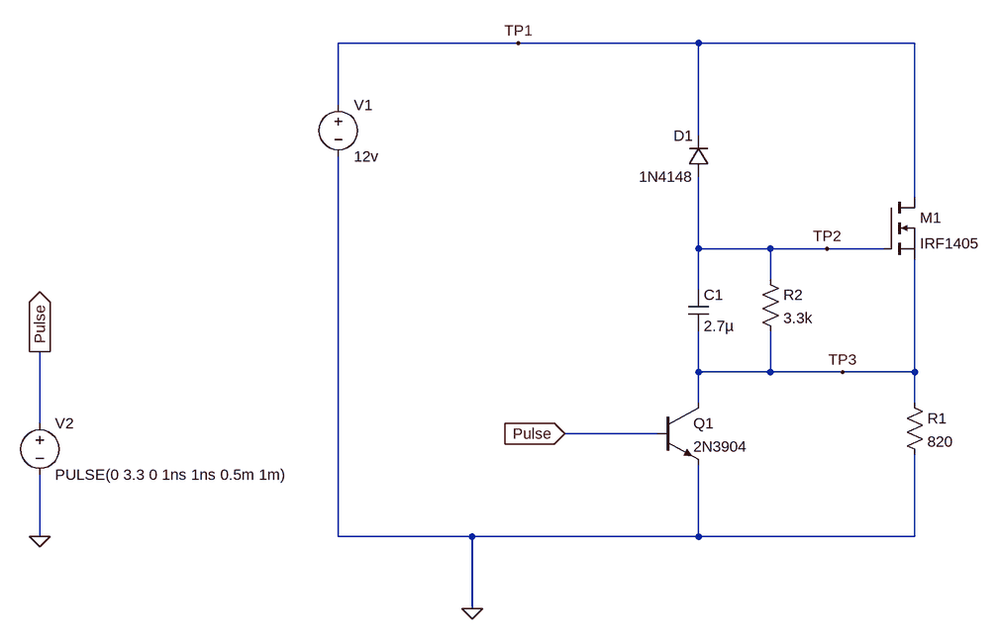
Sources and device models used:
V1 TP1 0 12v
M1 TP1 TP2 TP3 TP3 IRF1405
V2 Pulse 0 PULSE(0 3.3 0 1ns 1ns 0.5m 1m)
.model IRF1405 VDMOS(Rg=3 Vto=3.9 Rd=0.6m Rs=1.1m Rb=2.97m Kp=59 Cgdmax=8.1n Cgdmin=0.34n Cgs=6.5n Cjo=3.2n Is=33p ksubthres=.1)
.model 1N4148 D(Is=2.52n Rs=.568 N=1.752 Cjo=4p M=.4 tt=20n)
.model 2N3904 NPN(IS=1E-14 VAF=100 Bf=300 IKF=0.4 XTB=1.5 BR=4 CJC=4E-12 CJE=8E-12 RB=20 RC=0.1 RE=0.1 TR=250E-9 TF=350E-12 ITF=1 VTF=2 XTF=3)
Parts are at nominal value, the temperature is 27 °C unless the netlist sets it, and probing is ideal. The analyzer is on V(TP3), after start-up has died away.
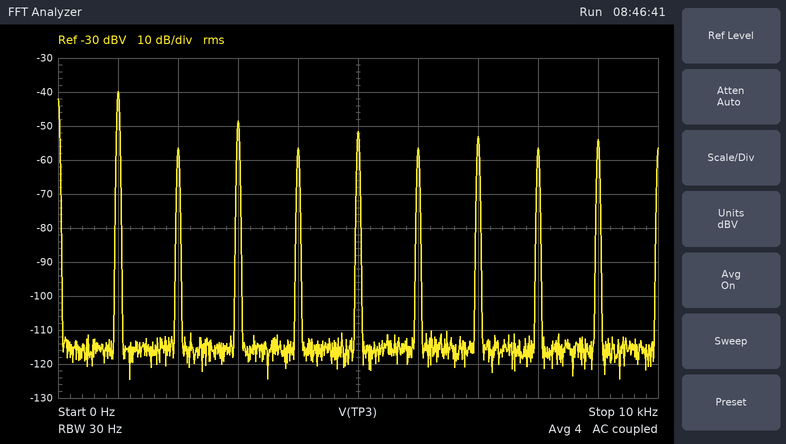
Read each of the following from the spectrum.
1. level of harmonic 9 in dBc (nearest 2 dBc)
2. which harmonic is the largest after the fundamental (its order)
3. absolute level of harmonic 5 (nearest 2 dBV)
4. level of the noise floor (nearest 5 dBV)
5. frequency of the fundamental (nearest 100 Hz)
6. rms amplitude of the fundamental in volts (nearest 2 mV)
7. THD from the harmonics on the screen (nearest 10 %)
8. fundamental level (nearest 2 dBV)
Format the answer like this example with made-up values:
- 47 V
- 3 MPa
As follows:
- -14 dBc
- 3
- -52 dBV
- -115 dBV
- 1.0 kHz
- 10 mV
- 60 %
- -40 dBV
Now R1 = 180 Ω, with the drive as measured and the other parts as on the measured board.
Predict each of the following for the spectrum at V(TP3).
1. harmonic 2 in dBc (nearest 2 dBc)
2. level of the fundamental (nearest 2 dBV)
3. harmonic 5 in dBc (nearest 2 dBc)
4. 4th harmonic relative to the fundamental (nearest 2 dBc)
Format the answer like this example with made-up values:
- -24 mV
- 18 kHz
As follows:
- -26 dBc
- -40 dBV
- -14 dBc
- -26 dBc
